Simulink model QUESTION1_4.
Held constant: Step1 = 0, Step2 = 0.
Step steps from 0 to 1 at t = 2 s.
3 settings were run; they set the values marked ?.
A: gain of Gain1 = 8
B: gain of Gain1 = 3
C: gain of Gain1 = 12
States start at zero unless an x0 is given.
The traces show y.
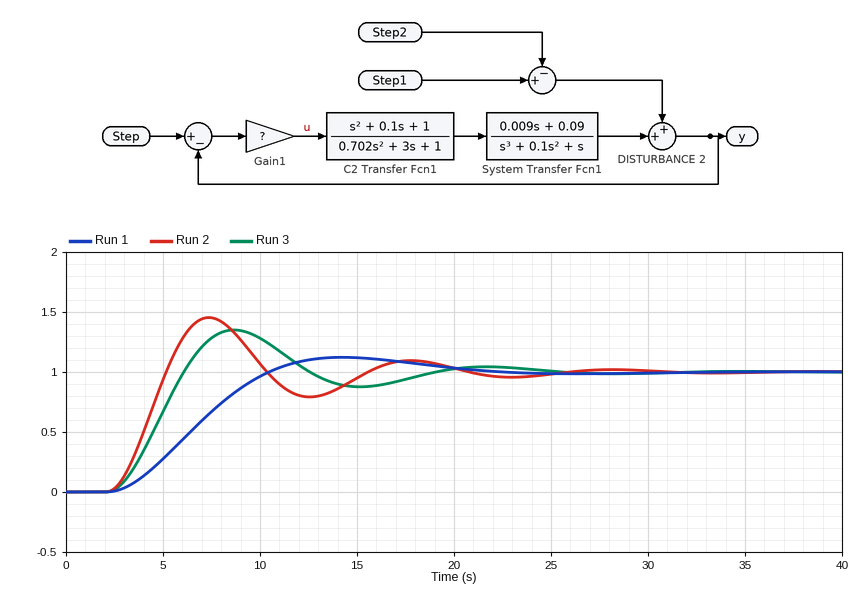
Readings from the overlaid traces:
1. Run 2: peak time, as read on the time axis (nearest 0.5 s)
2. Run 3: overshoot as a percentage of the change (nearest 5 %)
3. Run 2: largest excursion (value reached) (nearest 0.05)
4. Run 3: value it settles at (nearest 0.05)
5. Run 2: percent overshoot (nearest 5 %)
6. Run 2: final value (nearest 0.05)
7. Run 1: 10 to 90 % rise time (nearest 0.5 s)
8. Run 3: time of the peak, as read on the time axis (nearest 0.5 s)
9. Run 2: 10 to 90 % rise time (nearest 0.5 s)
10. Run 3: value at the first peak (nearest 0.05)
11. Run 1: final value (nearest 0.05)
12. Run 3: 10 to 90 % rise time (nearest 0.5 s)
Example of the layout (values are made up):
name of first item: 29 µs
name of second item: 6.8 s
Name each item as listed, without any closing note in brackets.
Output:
Run 2: peak time, as read on the time axis: 7.5 s
Run 3: overshoot as a percentage of the change: 35 %
Run 2: largest excursion (value reached): 1.45
Run 3: value it settles at: 1.00
Run 2: percent overshoot: 45 %
Run 2: final value: 1.00
Run 1: 10 to 90 % rise time: 5.5 s
Run 3: time of the peak, as read on the time axis: 8.5 s
Run 2: 10 to 90 % rise time: 2.0 s
Run 3: value at the first peak: 1.35
Run 1: final value: 1.00
Run 3: 10 to 90 % rise time: 2.5 s
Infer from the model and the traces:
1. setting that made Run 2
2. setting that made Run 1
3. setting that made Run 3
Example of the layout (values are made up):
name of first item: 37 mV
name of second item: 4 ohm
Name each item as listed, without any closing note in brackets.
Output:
setting that made Run 2: C
setting that made Run 1: B
setting that made Run 3: A
